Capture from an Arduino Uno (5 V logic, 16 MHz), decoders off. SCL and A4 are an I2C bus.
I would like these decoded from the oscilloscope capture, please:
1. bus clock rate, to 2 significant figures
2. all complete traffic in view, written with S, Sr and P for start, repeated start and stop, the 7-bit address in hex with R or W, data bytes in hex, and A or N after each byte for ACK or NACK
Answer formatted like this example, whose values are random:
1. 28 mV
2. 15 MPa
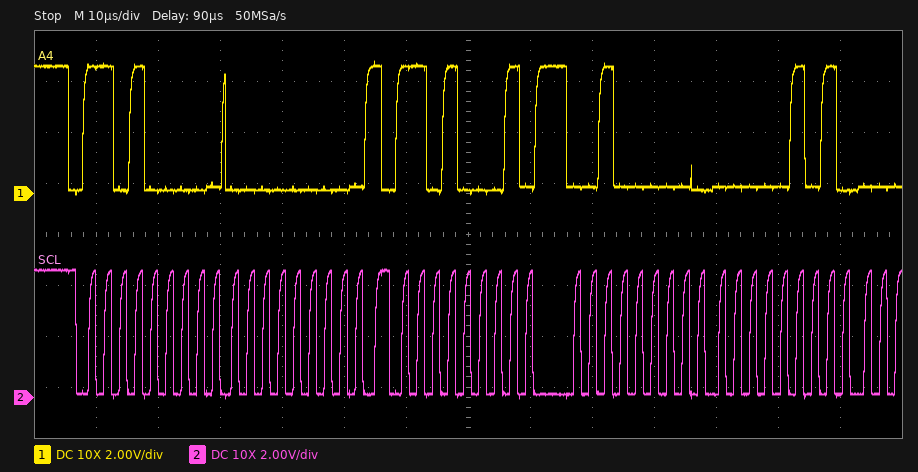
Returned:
1. 400 kHz
2. S 68W A 00 A Sr 68R A 20 A 05 A
